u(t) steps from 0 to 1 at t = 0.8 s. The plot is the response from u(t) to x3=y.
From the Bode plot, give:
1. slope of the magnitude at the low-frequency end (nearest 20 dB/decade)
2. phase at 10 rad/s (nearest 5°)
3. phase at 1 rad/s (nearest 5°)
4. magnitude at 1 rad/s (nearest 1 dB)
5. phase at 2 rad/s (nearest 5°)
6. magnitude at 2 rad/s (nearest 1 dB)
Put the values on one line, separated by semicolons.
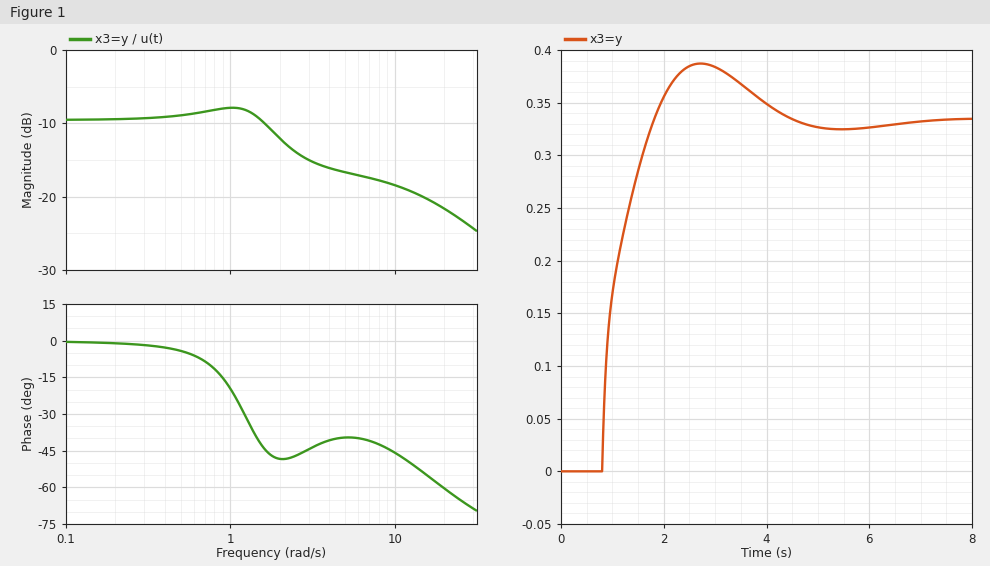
0 dB/decade; -45°; -20°; -8 dB; -50°; -12 dB
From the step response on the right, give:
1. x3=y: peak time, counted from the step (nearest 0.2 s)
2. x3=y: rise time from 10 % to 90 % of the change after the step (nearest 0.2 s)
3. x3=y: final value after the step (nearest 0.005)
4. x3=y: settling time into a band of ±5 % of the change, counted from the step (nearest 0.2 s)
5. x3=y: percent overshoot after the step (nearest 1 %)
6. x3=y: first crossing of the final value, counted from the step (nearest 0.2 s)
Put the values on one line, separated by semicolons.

2.0 s; 0.8 s; 0.335; 3.2 s; 16 %; 1.0 s
